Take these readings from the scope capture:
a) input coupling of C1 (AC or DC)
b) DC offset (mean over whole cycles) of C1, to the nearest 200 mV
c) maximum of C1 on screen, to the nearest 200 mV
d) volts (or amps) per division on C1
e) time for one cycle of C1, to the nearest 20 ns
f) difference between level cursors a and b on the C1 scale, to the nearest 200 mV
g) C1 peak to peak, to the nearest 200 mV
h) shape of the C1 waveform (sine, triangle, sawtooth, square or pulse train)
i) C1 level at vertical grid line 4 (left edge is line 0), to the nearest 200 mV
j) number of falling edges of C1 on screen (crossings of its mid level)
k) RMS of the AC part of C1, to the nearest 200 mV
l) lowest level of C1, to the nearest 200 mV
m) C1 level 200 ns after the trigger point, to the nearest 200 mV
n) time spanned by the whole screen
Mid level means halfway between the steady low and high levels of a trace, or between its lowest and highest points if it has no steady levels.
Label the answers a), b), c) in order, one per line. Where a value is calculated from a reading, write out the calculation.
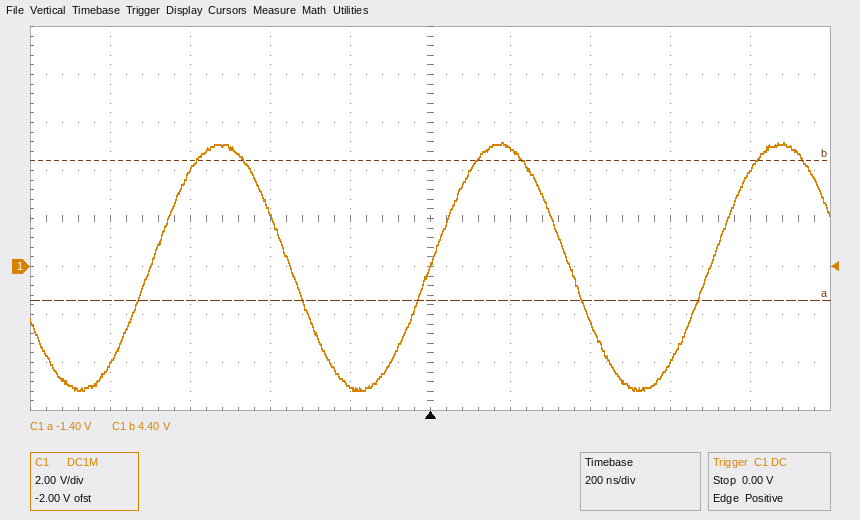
a) DC
b) (5.2 V + (-5.2 V)) / 2 ≈ 0.0 V
c) 5.2 V
d) 2 V
e) 700 ns
f) 5.8 V
g) 5.2 V − (-5.2 V) = 10.4 V
h) sine
i) -5.0 V
j) 2
k) 10.4 V / (2√2) ≈ 3.68 V, so 3.6 V to the nearest 200 mV
l) -5.2 V
m) 5.0 V
n) 2 µs
